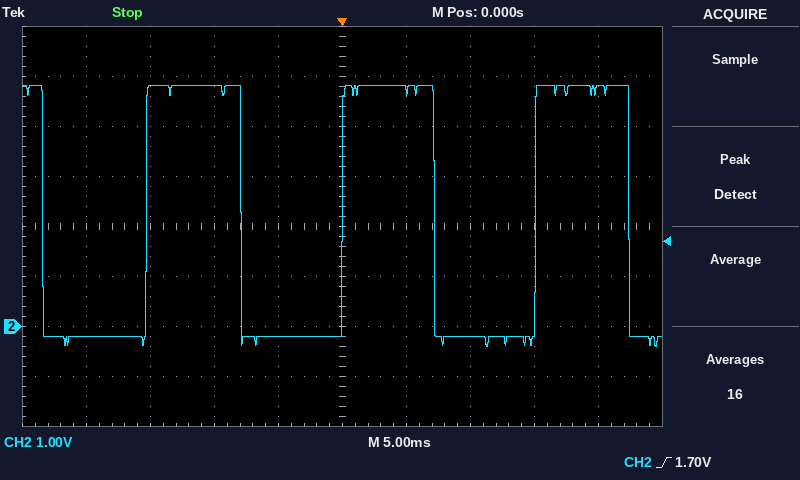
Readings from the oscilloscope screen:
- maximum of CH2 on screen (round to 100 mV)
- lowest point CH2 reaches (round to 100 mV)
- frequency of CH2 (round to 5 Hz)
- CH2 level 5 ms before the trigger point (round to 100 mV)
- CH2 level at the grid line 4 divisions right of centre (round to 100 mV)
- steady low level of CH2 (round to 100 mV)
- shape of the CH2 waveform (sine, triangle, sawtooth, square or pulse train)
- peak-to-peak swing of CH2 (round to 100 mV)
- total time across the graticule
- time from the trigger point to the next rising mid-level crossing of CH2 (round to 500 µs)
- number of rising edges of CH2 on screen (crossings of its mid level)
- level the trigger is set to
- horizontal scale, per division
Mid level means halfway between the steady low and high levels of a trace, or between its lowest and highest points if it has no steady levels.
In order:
4.8 V
-400 mV
65 Hz
-200 mV
4.7 V
-200 mV
square
5.2 V
50 ms
15.0 ms
3
1.70 V
5 ms
